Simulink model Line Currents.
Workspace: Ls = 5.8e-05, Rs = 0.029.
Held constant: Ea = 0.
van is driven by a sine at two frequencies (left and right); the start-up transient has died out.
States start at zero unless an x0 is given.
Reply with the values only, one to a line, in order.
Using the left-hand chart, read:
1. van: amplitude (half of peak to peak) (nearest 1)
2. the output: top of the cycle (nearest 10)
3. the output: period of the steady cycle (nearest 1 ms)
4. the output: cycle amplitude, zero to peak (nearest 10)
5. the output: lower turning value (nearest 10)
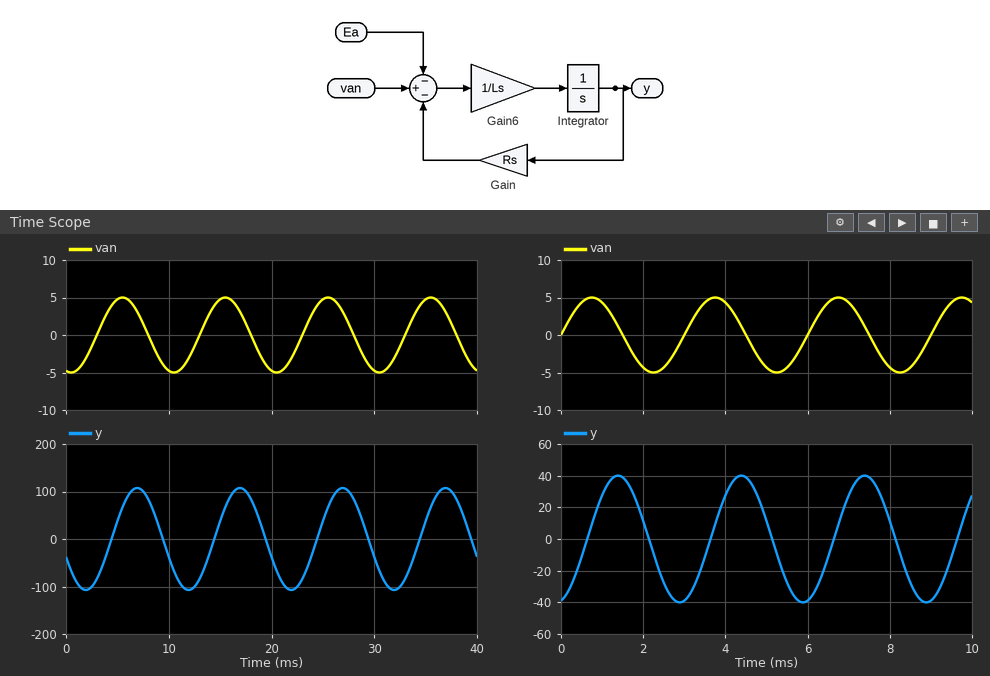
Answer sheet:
5
110
10 ms
110
-110
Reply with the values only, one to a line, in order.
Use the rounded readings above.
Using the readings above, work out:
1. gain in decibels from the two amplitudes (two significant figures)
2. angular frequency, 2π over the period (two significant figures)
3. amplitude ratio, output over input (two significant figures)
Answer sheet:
27 dB
0.63 rad/ms
22
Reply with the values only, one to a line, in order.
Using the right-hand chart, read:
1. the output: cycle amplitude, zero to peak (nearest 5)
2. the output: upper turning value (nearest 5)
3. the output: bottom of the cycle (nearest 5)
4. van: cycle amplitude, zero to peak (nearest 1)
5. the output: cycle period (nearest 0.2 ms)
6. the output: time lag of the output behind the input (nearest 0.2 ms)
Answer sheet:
40
40
-40
5
3.0 ms
0.6 ms
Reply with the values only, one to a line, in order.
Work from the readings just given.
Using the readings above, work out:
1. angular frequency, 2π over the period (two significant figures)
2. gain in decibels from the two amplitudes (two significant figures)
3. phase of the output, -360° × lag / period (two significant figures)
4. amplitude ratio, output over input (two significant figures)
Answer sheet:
2.1 rad/ms
18 dB
-72°
8.0
